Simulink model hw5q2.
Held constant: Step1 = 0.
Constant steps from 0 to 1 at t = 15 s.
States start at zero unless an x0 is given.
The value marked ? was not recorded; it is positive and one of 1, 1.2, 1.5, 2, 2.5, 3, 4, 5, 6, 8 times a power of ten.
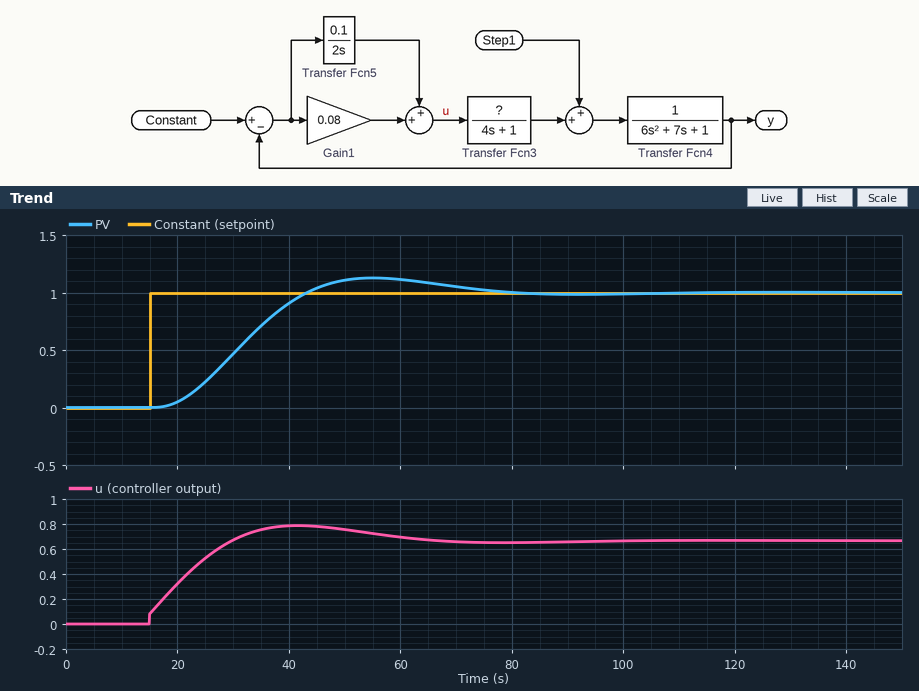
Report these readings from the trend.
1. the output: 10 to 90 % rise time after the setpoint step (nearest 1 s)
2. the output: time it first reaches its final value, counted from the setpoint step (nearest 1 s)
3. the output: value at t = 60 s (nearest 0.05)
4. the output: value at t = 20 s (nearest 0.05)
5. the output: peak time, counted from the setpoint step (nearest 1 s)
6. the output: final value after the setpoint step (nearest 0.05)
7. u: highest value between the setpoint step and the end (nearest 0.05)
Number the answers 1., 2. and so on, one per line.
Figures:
1. 18 s
2. 28 s
3. 1.10
4. 0.05
5. 40 s
6. 1.00
7. 0.80
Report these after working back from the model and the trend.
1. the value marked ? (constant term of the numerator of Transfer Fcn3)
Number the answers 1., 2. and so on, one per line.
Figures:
1. 1.5
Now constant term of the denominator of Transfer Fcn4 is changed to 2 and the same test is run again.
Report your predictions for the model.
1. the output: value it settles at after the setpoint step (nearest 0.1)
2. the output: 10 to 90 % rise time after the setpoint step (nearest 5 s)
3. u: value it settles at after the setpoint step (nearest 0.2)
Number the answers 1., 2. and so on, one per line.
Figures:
1. 1.0
2. 45 s
3. 1.4
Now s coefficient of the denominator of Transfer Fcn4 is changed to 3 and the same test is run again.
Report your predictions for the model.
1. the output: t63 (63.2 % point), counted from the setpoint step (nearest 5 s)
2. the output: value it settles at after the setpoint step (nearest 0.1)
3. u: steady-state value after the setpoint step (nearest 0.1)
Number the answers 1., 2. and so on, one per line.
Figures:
1. 15 s
2. 1.0
3. 0.7
